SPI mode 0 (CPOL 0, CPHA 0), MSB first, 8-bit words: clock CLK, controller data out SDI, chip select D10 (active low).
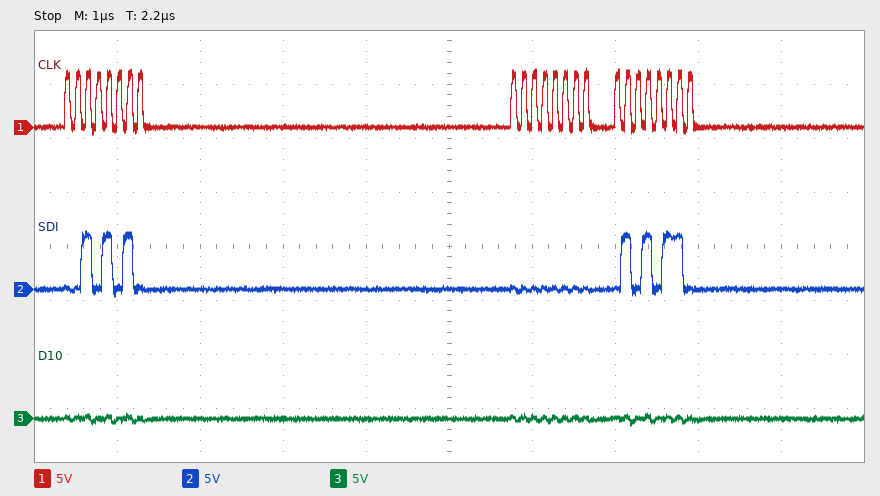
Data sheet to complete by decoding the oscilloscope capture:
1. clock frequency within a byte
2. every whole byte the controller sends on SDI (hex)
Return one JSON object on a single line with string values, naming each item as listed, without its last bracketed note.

{"clock frequency within a byte": "8 MHz", "every whole byte the controller sends on SDI": "2A 00 56"}
